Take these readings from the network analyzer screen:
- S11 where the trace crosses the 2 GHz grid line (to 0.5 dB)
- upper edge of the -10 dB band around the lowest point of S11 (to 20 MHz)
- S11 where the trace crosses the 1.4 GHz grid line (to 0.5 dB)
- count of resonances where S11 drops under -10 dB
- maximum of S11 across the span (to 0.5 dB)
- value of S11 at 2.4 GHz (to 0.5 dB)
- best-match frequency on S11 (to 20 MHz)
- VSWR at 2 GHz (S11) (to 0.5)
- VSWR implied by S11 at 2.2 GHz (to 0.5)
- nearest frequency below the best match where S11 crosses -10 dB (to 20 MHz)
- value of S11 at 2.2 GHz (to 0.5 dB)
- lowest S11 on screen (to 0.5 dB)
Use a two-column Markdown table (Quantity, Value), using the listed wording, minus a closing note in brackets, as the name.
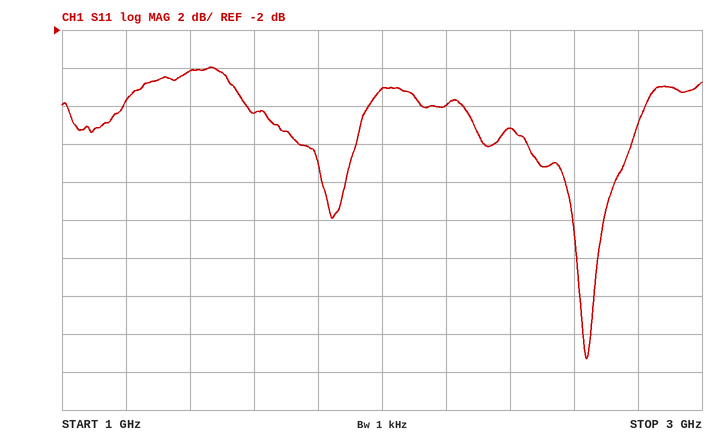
| Quantity | Value |
|---|---|
| S11 where the trace crosses the 2 GHz grid line | -5.0 dB |
| upper edge of the -10 dB band around the lowest point of S11 | 2.72 GHz |
| S11 where the trace crosses the 1.4 GHz grid line | -4.0 dB |
| count of resonances where S11 drops under -10 dB | 2 |
| maximum of S11 across the span | -4.0 dB |
| value of S11 at 2.4 GHz | -7.0 dB |
| best-match frequency on S11 | 2.64 GHz |
| VSWR at 2 GHz (S11) | 3.5 |
| VSWR implied by S11 at 2.2 GHz | 3.0 |
| nearest frequency below the best match where S11 crosses -10 dB | 2.58 GHz |
| value of S11 at 2.2 GHz | -6.0 dB |
| lowest S11 on screen | -19.5 dB |
